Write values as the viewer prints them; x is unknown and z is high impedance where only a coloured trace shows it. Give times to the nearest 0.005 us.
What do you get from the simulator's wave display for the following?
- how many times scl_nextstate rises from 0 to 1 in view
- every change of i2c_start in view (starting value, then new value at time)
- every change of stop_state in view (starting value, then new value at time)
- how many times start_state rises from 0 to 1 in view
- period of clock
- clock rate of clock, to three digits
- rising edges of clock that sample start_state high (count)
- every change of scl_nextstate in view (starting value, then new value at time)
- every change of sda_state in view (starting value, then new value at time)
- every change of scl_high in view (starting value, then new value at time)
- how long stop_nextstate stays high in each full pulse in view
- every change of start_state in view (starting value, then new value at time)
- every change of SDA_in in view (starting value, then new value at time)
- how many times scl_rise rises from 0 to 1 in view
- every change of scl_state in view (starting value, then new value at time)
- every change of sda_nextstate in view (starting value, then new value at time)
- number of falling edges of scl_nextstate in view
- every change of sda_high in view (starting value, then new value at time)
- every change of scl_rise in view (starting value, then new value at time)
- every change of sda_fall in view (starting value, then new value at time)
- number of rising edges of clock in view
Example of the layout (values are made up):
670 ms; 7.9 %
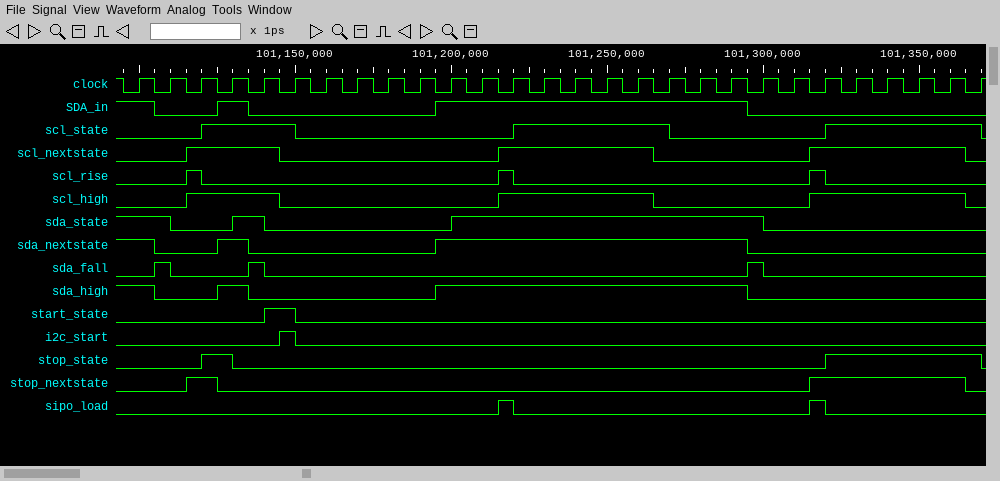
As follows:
3; 0, 1 at 101.145 us, 0 at 101.15 us; 0, 1 at 101.12 us, 0 at 101.13 us, 1 at 101.32 us, 0 at 101.37 us; 1; 0.01 us; 100 MHz; 1; 0, 1 at 101.115 us, 0 at 101.145 us, 1 at 101.215 us, 0 at 101.265 us, 1 at 101.315 us, 0 at 101.365 us; 1, 0 at 101.11 us, 1 at 101.13 us, 0 at 101.14 us, 1 at 101.2 us, 0 at 101.3 us; 0, 1 at 101.115 us, 0 at 101.145 us, 1 at 101.215 us, 0 at 101.265 us, 1 at 101.315 us, 0 at 101.365 us; 0.01 us, 0.05 us; 0, 1 at 101.14 us, 0 at 101.15 us; 1, 0 at 101.105 us, 1 at 101.125 us, 0 at 101.135 us, 1 at 101.195 us, 0 at 101.295 us; 3; 0, 1 at 101.12 us, 0 at 101.15 us, 1 at 101.22 us, 0 at 101.27 us, 1 at 101.32 us, 0 at 101.37 us; 1, 0 at 101.105 us, 1 at 101.125 us, 0 at 101.135 us, 1 at 101.195 us, 0 at 101.295 us; 3; 1, 0 at 101.105 us, 1 at 101.125 us, 0 at 101.135 us, 1 at 101.195 us, 0 at 101.295 us; 0, 1 at 101.115 us, 0 at 101.12 us, 1 at 101.215 us, 0 at 101.22 us, 1 at 101.315 us, 0 at 101.32 us; 0, 1 at 101.105 us, 0 at 101.11 us, 1 at 101.135 us, 0 at 101.14 us, 1 at 101.295 us, 0 at 101.3 us; 28
